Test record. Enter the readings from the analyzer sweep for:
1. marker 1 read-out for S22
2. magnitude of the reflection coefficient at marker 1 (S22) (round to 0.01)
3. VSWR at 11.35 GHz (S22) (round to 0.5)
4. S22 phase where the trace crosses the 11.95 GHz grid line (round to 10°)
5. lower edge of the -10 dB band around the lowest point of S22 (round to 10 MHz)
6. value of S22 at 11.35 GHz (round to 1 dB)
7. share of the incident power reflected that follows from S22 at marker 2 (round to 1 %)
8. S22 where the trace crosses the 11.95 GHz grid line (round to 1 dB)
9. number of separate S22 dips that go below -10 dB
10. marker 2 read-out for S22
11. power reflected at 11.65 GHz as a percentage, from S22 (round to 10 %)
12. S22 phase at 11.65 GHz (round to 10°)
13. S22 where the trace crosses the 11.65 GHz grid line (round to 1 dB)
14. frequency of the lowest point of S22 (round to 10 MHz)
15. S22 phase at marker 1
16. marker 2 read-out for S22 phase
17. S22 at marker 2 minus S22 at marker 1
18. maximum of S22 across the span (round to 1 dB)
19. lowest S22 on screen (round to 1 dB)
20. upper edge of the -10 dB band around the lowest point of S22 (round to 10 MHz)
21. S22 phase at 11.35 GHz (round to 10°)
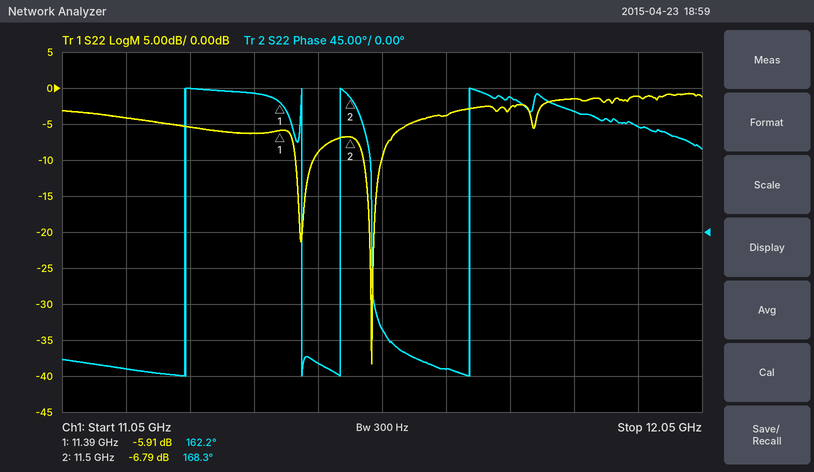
-5.91 dB
0.51
3.0
130°
11.52 GHz
-6 dB
21 %
-1 dB
2
-6.79 dB
40 %
-170°
-4 dB
11.53 GHz
162.2°
168.3°
-0.88 dB
-1 dB
-38 dB
11.55 GHz
170°
